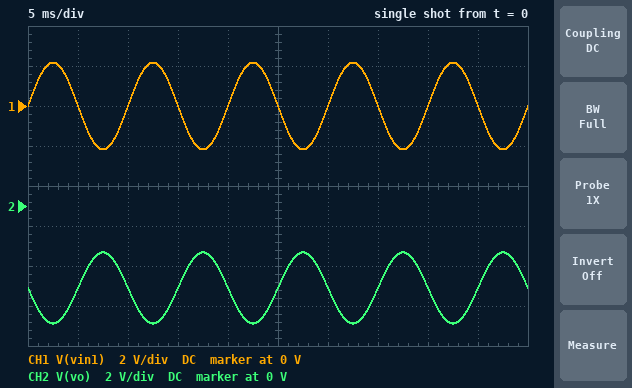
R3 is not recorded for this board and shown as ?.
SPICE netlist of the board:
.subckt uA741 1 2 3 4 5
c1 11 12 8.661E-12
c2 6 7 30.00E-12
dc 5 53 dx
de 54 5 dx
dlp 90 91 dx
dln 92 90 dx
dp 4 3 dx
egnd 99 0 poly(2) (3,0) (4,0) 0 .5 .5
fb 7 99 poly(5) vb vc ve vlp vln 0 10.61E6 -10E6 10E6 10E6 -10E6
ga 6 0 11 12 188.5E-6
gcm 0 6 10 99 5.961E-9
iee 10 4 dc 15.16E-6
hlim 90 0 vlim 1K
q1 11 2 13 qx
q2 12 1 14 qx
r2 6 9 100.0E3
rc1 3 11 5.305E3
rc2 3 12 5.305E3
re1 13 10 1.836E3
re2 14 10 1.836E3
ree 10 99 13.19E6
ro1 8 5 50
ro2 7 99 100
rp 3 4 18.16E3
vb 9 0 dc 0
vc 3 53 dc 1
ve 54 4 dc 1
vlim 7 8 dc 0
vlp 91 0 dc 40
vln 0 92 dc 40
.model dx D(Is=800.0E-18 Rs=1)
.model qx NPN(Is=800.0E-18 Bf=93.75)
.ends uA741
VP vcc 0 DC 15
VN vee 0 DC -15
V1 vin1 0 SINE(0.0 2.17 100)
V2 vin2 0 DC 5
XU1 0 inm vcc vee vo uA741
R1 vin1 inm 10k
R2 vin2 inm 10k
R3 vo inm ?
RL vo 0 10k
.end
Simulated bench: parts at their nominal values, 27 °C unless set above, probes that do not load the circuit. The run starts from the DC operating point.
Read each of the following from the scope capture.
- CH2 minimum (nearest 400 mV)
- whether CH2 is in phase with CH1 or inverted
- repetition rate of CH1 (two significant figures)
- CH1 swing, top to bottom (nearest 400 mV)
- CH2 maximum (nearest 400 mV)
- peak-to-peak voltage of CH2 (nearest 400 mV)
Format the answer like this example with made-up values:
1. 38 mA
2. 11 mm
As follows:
1. -6.0 V
2. inverted
3. 100 Hz
4. 4.4 V
5. -2.4 V
6. 3.6 V
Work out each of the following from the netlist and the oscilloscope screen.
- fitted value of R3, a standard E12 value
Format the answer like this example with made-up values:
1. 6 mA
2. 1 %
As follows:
1. 8.2 kΩ
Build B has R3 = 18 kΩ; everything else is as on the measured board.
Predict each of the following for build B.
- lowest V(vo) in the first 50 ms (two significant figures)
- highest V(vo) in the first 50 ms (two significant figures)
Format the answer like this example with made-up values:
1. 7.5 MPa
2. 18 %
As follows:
1. -13 V
2. -5.1 V
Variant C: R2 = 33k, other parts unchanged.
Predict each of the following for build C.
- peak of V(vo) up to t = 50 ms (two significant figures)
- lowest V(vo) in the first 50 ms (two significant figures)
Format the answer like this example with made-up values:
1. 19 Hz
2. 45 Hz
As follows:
1. 540 mV
2. -3.0 V
